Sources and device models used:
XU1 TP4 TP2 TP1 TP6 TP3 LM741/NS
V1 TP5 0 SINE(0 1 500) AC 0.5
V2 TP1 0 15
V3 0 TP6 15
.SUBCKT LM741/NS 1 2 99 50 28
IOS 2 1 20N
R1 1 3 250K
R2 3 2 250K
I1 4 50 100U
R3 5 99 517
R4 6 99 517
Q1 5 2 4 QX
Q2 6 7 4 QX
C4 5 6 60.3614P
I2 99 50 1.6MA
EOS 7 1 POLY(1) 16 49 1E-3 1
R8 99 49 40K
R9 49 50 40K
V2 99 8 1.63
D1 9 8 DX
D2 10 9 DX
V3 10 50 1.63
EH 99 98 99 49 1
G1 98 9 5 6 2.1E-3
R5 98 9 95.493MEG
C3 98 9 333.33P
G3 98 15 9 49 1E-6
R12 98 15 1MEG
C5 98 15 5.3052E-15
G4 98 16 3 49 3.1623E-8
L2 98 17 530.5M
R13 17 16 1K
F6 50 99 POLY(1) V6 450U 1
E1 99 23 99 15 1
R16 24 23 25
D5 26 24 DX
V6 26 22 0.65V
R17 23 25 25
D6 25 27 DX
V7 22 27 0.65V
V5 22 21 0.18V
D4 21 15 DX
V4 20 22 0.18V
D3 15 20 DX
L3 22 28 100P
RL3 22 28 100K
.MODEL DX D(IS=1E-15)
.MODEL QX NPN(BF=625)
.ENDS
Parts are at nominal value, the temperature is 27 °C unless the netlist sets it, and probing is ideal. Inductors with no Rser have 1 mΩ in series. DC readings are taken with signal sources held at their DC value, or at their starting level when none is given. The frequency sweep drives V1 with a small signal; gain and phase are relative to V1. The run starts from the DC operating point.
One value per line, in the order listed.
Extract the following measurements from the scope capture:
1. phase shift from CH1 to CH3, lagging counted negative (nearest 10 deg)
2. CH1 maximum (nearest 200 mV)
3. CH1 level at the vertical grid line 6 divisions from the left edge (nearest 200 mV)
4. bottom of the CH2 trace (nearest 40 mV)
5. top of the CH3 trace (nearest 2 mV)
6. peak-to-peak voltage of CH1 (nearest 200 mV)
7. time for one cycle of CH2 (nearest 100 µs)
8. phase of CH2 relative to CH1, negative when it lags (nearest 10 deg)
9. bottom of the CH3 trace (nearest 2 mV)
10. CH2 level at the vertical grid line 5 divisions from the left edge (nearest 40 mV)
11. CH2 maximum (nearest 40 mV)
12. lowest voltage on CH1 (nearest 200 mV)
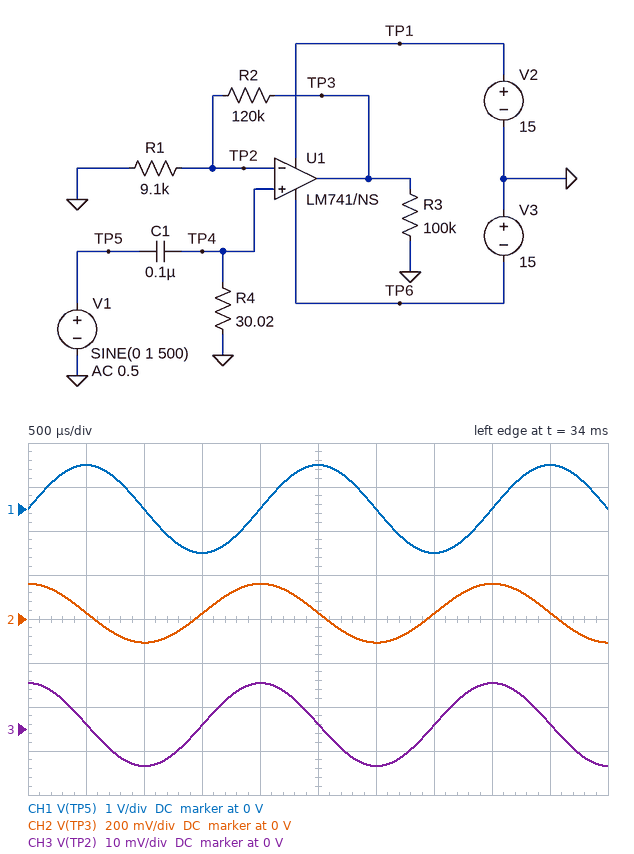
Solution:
90 deg
1.0 V
0 V
-120 mV
10 mV
2.0 V
2.0 ms
90 deg
-8 mV
40 mV
160 mV
-1.0 V
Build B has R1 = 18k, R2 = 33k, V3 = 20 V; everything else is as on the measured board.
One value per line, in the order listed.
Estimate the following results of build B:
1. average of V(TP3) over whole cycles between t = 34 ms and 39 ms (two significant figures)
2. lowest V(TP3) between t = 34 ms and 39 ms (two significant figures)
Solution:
6.4 mV
-20 mV
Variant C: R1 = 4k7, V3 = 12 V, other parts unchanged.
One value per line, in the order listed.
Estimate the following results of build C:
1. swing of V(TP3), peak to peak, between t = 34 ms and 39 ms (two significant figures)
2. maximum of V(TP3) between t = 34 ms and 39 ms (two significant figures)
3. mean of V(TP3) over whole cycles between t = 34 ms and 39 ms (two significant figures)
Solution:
500 mV
290 mV
38 mV
